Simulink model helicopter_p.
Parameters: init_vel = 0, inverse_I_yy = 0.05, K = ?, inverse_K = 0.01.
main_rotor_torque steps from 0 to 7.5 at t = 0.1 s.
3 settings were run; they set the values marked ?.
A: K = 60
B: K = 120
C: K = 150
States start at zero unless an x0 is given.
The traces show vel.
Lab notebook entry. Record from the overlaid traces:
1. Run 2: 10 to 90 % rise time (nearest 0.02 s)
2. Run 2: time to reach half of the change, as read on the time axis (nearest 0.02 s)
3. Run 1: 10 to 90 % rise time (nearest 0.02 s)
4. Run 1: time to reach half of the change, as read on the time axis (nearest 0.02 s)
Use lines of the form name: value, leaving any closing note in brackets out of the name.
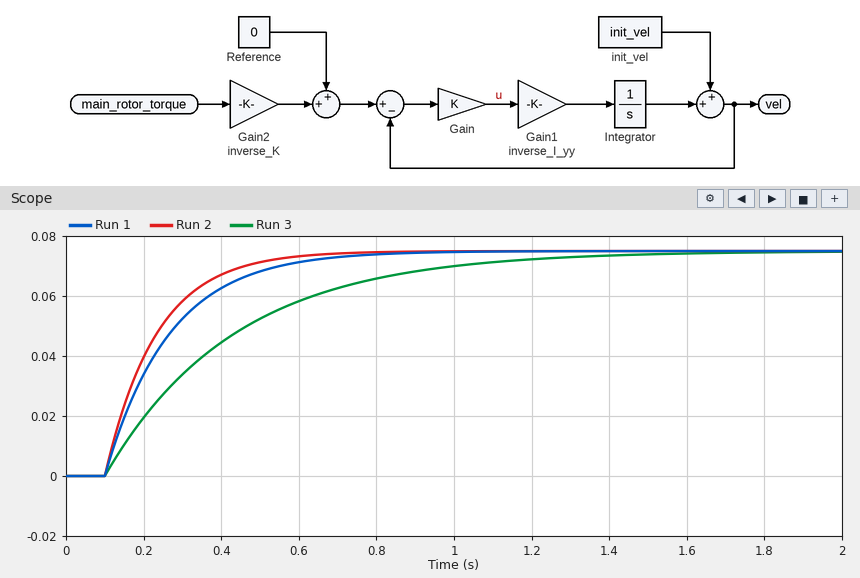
Run 2: 10 to 90 % rise time: 0.30 s
Run 2: time to reach half of the change, as read on the time axis: 0.20 s
Run 1: 10 to 90 % rise time: 0.36 s
Run 1: time to reach half of the change, as read on the time axis: 0.22 s
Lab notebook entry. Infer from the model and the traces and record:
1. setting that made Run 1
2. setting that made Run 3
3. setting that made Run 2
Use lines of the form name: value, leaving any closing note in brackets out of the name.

setting that made Run 1: B
setting that made Run 3: A
setting that made Run 2: C
